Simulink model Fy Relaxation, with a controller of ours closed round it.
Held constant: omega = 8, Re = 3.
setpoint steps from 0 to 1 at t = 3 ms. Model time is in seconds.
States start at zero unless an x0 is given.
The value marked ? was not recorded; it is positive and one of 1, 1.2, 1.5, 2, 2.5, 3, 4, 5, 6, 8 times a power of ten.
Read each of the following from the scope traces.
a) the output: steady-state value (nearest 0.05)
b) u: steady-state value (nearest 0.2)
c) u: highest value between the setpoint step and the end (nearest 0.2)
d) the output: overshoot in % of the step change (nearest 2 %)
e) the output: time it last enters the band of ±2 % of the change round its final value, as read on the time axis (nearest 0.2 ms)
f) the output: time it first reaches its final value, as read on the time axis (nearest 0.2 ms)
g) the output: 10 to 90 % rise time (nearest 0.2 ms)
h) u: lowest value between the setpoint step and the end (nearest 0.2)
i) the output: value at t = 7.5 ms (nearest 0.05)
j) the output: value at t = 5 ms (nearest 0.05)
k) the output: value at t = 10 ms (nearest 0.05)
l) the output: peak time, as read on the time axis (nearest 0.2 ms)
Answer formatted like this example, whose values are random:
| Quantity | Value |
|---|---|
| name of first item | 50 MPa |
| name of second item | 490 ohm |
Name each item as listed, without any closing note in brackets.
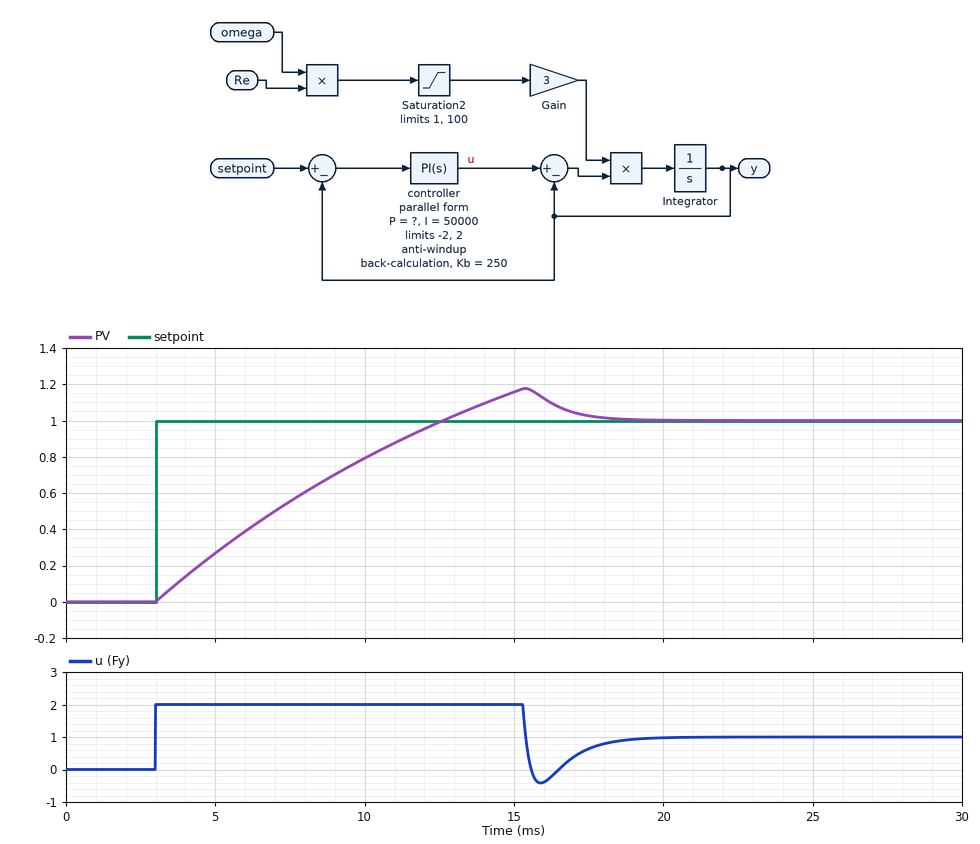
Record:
| Quantity | Value |
|---|---|
| the output: steady-state value | 1.00 |
| u: steady-state value | 1.0 |
| u: highest value between the setpoint step and the end | 2.0 |
| the output: overshoot in % of the step change | 18 % |
| the output: time it last enters the band of ±2 % of the change round its final value, as read on the time axis | 17.8 ms |
| the output: time it first reaches its final value, as read on the time axis | 12.6 ms |
| the output: 10 to 90 % rise time | 7.6 ms |
| u: lowest value between the setpoint step and the end | -0.4 |
| the output: value at t = 7.5 ms | 0.55 |
| the output: value at t = 5 ms | 0.25 |
| the output: value at t = 10 ms | 0.80 |
| the output: peak time, as read on the time axis | 15.4 ms |
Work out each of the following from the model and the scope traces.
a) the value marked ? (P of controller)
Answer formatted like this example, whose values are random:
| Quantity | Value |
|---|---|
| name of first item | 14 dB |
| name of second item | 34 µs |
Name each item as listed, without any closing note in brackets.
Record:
| Quantity | Value |
|---|---|
| the value marked ? | 60 |
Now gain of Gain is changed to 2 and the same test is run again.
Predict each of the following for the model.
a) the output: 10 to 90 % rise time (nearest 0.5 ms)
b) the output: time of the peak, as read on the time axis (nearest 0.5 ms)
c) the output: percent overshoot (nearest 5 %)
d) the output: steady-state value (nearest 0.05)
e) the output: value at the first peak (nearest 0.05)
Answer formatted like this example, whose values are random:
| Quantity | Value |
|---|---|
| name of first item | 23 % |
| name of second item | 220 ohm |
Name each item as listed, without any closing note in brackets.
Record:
| Quantity | Value |
|---|---|
| the output: 10 to 90 % rise time | 11.5 ms |
| the output: time of the peak, as read on the time axis | 20.5 ms |
| the output: percent overshoot | 15 % |
| the output: steady-state value | 1.00 |
| the output: value at the first peak | 1.15 |
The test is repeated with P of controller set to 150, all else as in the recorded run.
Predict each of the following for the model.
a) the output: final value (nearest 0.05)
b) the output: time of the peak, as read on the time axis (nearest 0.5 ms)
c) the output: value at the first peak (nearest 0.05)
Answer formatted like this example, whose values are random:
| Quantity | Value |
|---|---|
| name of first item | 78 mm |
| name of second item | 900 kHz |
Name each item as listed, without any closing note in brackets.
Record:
| Quantity | Value |
|---|---|
| the output: final value | 1.00 |
| the output: time of the peak, as read on the time axis | 13.5 ms |
| the output: value at the first peak | 1.05 |
